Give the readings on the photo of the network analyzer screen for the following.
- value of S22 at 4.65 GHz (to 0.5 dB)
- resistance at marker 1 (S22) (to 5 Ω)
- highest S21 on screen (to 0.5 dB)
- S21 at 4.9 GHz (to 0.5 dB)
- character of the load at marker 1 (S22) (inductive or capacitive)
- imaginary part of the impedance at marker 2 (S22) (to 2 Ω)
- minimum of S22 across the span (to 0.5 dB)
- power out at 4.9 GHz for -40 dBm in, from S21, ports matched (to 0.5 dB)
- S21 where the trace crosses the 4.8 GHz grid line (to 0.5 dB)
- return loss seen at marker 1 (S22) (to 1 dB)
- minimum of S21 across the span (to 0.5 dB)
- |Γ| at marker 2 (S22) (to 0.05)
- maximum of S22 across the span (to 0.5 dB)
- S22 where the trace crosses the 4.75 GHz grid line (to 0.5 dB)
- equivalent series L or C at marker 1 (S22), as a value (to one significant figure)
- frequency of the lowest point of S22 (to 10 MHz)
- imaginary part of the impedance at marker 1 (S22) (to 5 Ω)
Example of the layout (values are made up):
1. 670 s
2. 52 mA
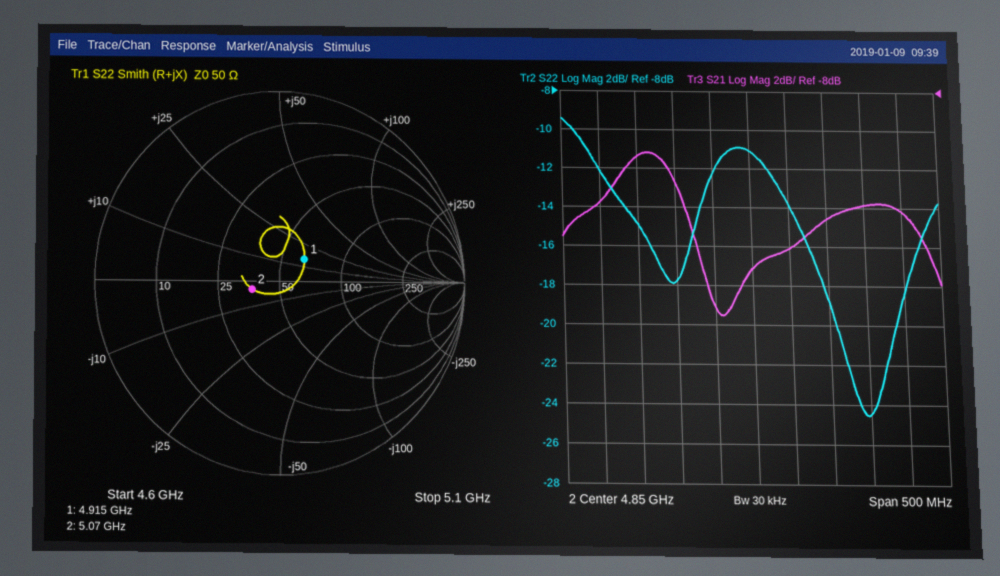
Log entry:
1. -12.0 dB
2. 65 Ω
3. -11.0 dB
4. -16.0 dB
5. inductive
6. -4 Ω
7. -24.5 dB
8. -56.0 dBm
9. -19.0 dB
10. 15 dB
11. -19.5 dB
12. 0.15
13. -9.5 dB
14. -18.0 dB
15. 500 pH
16. 5.00 GHz
17. +15 Ω
